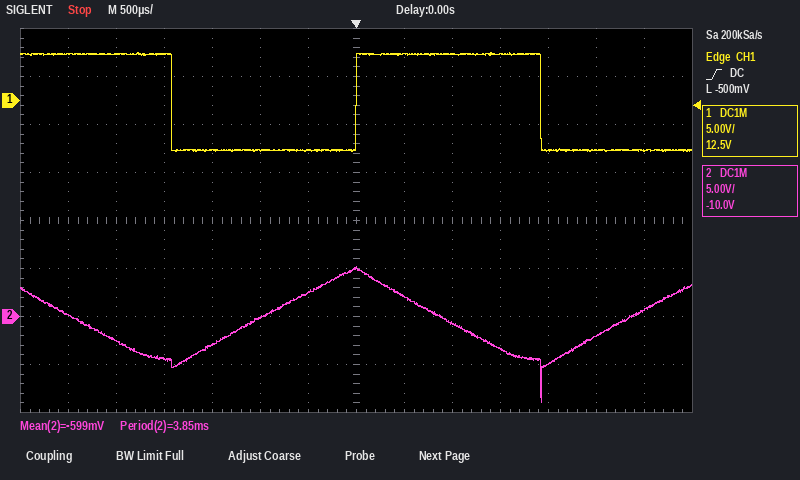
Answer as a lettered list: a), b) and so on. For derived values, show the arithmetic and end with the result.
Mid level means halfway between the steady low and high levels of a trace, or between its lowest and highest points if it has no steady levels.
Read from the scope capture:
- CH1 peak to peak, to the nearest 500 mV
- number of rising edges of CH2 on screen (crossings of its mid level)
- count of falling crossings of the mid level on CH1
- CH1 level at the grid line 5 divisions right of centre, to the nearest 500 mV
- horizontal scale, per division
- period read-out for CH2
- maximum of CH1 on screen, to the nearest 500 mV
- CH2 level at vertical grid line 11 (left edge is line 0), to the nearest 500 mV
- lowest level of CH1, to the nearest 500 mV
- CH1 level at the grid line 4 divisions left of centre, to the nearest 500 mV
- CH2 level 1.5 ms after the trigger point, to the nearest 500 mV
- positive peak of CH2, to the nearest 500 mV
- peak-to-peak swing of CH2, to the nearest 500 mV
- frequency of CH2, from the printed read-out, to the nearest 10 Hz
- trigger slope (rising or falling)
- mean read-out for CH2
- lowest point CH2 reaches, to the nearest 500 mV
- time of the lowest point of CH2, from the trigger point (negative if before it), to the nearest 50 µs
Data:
a) 5.0 V − (-5.5 V) = 10.5 V
b) 2
c) 2
d) -5.0 V
e) 500 µs
f) 3.85 ms
g) 5.0 V
h) -5.0 V
i) -5.5 V
j) 5.0 V
k) -3.5 V
l) 5.0 V
m) 5.0 V − (-9.0 V) = 14.0 V
n) 1 / 3.85 ms ≈ 260 Hz
o) rising
p) -599 mV
q) -9.0 V
r) +1.95 ms
